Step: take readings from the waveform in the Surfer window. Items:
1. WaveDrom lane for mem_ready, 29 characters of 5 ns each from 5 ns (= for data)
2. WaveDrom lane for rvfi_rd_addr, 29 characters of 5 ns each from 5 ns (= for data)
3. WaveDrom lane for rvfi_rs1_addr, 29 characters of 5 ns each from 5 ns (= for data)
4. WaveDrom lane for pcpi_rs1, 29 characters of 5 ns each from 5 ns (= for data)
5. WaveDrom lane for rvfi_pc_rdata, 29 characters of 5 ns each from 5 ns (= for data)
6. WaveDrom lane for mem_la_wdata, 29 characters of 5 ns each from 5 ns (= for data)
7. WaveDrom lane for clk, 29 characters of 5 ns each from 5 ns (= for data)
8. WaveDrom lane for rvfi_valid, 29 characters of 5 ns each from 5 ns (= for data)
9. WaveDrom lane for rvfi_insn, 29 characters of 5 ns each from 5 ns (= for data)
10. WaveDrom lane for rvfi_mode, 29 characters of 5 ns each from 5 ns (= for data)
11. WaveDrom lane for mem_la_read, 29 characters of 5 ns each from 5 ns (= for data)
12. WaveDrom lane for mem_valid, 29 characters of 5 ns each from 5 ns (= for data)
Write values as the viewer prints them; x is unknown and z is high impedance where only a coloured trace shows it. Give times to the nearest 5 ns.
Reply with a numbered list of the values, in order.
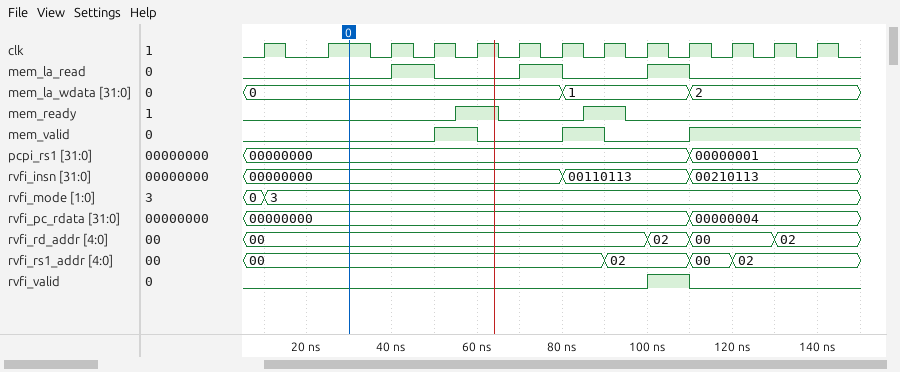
1. {name: 'mem_ready', wave: '0.........1.0...1.0..........'}
2. {name: 'rvfi_rd_addr', wave: '=..................=.=...=...', data: '00 02 00 02'}
3. {name: 'rvfi_rs1_addr', wave: '=................=...=.=.....', data: '00 02 00 02'}
4. {name: 'pcpi_rs1', wave: '=....................=.......', data: '00000000 00000001'}
5. {name: 'rvfi_pc_rdata', wave: '=....................=.......', data: '00000000 00000004'}
6. {name: 'mem_la_wdata', wave: '=..............=.....=.......', data: '0 1 2'}
7. {name: 'clk', wave: '010.1.01010101010101010101010'}
8. {name: 'rvfi_valid', wave: '0..................1.0.......'}
9. {name: 'rvfi_insn', wave: '=..............=.....=.......', data: '00000000 00110113 00210113'}
10. {name: 'rvfi_mode', wave: '==...........................', data: '0 3'}
11. {name: 'mem_la_read', wave: '0......1.0...1.0...1.0.......'}
12. {name: 'mem_valid', wave: '0........1.0...1.0...1.......'}
